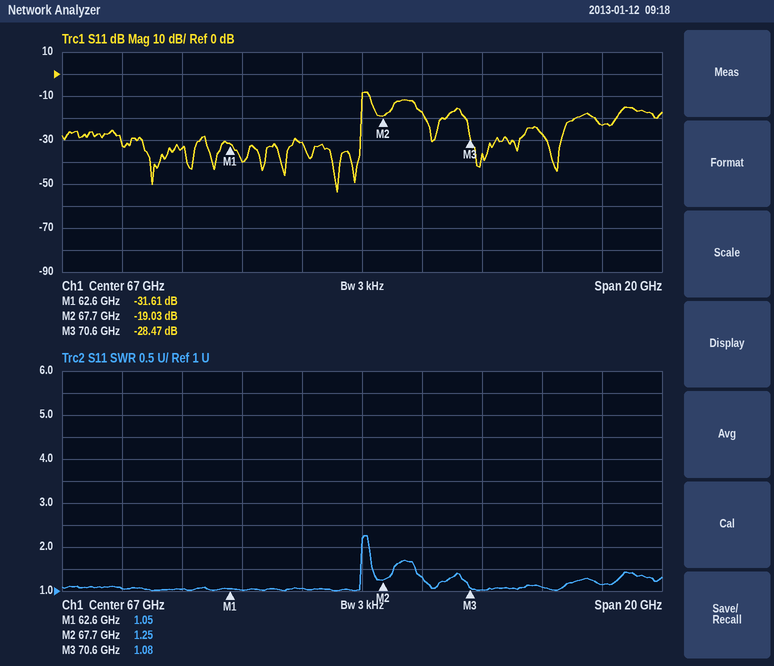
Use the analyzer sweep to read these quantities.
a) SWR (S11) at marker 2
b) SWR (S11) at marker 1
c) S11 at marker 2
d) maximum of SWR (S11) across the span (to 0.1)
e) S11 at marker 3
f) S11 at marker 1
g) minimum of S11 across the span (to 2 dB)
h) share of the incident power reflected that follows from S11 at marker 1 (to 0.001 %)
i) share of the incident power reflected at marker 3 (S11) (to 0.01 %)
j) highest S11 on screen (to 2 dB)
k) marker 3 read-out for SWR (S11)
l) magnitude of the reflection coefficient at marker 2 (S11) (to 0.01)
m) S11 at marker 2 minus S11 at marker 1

1.25
1.05
-19.03 dB
2.3
-28.47 dB
-31.61 dB
-54 dB
0.069 %
0.14 %
-8 dB
1.08
0.11
12.58 dB
